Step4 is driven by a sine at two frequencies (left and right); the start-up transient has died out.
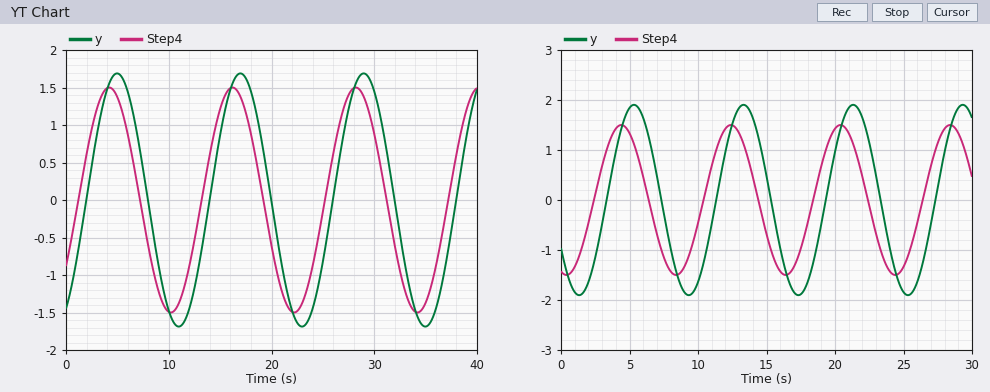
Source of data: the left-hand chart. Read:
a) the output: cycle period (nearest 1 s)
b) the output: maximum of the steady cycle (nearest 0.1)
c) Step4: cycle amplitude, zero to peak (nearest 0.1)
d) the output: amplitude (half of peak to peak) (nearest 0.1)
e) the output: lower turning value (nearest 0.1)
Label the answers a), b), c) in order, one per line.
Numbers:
a) 12 s
b) 1.7
c) 1.5
d) 1.7
e) -1.7
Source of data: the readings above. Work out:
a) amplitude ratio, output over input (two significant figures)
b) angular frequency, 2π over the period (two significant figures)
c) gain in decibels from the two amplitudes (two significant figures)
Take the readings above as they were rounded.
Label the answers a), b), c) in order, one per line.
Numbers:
a) 1.1
b) 0.52 rad/s
c) 1.1 dB
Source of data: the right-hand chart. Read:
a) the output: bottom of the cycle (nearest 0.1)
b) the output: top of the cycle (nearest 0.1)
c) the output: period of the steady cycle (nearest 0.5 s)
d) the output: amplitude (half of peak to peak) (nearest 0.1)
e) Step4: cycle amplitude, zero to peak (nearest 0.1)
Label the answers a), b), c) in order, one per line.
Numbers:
a) -1.9
b) 1.9
c) 8.0 s
d) 1.9
e) 1.5
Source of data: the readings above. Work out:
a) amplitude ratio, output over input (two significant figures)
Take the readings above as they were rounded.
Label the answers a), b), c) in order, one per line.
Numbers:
a) 1.3
